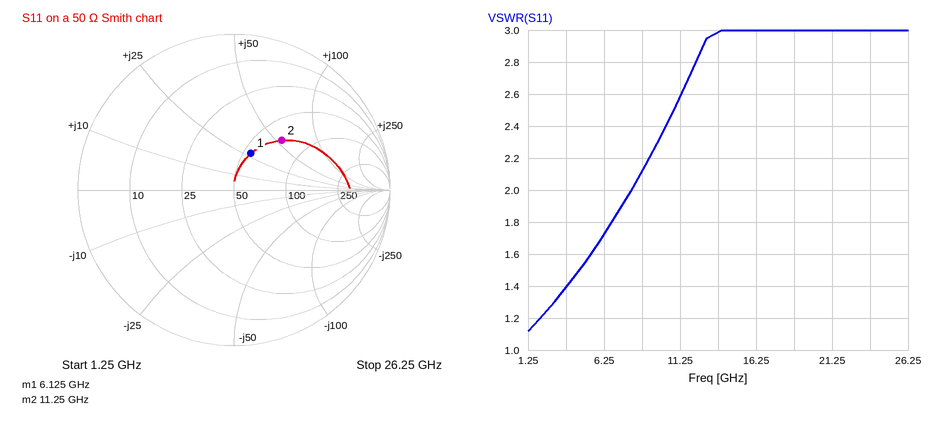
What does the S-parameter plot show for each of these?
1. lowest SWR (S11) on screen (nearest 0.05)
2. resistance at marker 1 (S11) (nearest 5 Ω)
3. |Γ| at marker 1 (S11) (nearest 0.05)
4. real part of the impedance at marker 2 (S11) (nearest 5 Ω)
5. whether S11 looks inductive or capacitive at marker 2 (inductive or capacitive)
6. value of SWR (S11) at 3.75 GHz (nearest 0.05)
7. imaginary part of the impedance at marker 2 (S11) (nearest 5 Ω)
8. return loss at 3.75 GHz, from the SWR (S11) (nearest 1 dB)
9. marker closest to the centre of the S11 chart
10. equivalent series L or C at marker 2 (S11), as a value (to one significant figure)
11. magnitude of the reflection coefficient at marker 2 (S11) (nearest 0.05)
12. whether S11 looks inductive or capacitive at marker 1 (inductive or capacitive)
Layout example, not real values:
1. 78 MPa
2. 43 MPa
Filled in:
1. 1.10
2. 55 Ω
3. 0.25
4. 70 Ω
5. inductive
6. 1.40
7. +55 Ω
8. 16 dB
9. marker 1
10. 800 pH
11. 0.45
12. inductive
